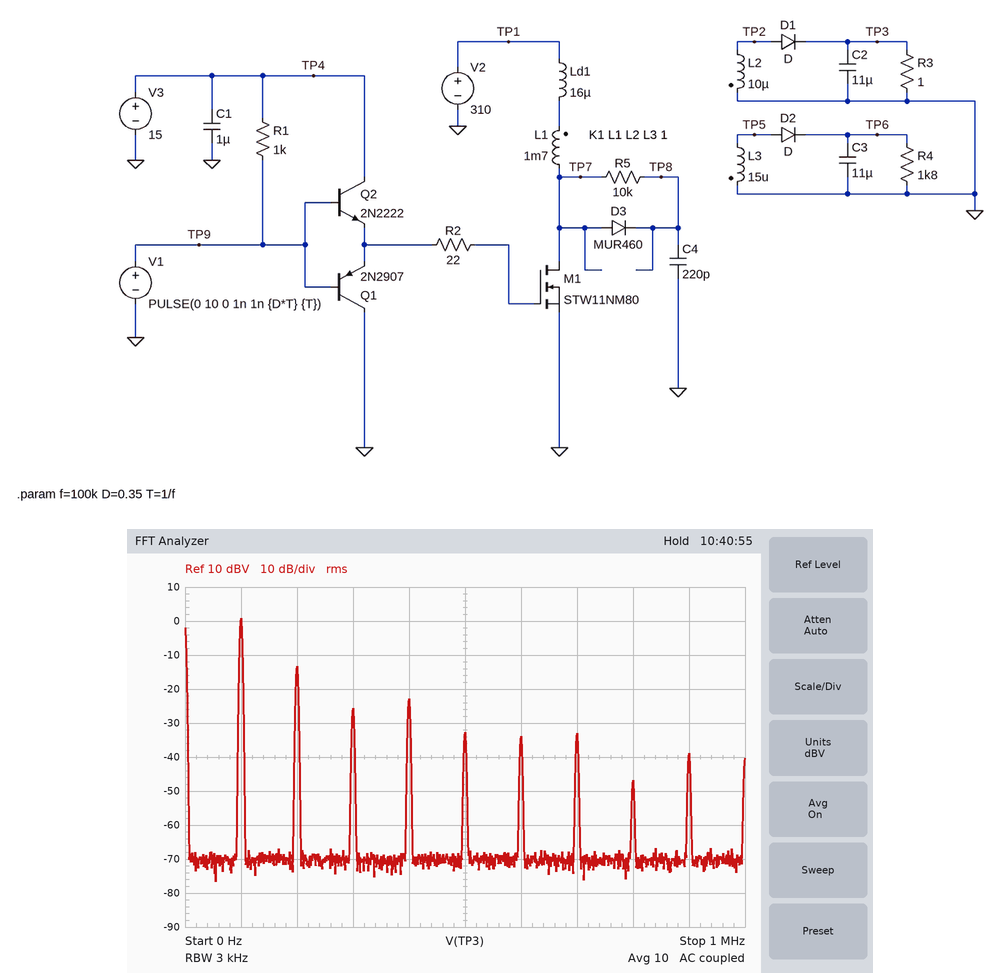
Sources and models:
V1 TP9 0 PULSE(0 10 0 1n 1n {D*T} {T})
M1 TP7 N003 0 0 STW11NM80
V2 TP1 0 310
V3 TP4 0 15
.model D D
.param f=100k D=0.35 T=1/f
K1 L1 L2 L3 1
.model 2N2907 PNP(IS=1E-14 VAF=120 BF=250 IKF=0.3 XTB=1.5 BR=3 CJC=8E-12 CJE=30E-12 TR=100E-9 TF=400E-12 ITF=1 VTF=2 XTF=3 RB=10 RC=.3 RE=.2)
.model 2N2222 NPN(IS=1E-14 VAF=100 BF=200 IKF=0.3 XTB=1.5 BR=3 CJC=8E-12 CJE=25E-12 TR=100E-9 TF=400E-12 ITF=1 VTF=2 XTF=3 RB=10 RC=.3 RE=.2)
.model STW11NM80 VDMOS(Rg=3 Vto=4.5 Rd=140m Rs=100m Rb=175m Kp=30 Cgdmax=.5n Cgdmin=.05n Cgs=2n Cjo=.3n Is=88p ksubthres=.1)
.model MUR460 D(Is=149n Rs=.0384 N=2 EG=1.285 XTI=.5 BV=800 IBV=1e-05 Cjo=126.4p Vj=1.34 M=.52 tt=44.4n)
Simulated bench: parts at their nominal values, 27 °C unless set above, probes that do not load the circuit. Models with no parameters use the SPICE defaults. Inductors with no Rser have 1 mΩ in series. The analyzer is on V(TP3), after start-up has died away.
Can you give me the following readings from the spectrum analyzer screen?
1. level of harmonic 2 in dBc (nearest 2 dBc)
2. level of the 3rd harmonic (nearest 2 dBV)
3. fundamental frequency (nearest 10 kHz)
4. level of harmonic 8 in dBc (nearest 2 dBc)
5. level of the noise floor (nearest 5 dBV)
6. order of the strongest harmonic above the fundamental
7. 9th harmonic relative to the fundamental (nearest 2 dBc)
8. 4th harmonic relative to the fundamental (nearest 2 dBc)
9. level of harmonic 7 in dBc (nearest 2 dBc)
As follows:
-14 dBc
-26 dBV
100 kHz
-48 dBc
-70 dBV
2
-40 dBc
-24 dBc
-34 dBc
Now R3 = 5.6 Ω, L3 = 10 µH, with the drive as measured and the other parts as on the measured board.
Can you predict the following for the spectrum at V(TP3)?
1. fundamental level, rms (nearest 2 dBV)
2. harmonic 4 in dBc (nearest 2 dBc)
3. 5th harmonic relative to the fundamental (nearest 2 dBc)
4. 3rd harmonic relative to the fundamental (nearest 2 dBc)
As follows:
-10 dBV
-26 dBc
-30 dBc
-20 dBc
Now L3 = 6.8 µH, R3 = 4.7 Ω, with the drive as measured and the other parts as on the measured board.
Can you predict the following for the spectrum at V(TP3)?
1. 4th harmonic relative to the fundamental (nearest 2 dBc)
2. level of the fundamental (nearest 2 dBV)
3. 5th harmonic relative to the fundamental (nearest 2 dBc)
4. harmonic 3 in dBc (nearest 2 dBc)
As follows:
-26 dBc
-10 dBV
-30 dBc
-20 dBc
